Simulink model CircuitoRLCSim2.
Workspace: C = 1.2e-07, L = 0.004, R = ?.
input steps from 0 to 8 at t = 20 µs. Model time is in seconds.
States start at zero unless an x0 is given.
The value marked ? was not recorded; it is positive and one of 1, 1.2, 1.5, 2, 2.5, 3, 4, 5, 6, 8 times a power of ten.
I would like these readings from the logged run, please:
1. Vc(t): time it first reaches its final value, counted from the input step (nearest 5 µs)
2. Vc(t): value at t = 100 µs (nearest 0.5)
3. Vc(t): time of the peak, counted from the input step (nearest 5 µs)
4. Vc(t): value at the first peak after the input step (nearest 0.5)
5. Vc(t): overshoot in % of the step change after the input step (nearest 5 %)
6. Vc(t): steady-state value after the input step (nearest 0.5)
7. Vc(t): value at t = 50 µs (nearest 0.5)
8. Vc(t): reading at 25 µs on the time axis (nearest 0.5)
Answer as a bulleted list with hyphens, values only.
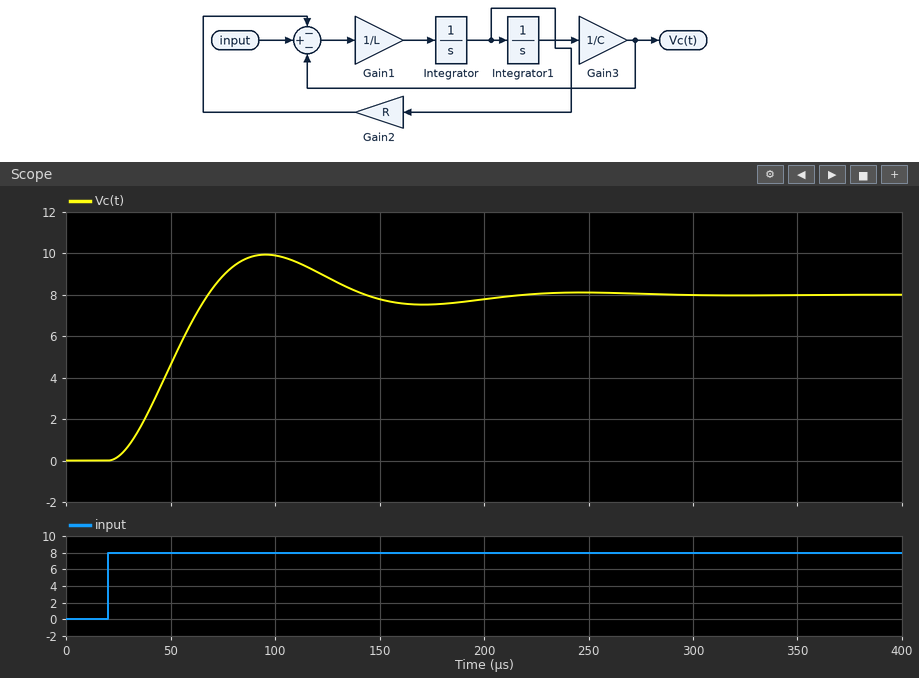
- 50 µs
- 10.0
- 75 µs
- 10.0
- 25 %
- 8.0
- 4.5
- 0.0
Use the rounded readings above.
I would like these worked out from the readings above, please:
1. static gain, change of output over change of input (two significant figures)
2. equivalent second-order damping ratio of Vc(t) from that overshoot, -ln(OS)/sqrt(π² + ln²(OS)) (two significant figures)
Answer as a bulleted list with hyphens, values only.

- 1.0
- 0.40
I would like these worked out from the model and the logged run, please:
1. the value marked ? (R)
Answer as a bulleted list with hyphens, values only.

- 150
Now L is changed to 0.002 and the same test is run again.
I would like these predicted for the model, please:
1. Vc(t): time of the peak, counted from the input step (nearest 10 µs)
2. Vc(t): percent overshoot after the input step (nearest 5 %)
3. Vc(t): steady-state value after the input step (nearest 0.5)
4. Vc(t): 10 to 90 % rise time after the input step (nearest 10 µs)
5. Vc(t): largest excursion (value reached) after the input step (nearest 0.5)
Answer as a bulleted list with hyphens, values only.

- 60 µs
- 10 %
- 8.0
- 30 µs
- 9.0
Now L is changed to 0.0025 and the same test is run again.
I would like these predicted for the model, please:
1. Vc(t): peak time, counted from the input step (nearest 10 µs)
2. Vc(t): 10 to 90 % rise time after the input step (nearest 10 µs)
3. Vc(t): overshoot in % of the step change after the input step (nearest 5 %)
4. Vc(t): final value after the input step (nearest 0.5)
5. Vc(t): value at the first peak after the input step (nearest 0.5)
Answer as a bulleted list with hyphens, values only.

- 60 µs
- 30 µs
- 15 %
- 8.0
- 9.0
